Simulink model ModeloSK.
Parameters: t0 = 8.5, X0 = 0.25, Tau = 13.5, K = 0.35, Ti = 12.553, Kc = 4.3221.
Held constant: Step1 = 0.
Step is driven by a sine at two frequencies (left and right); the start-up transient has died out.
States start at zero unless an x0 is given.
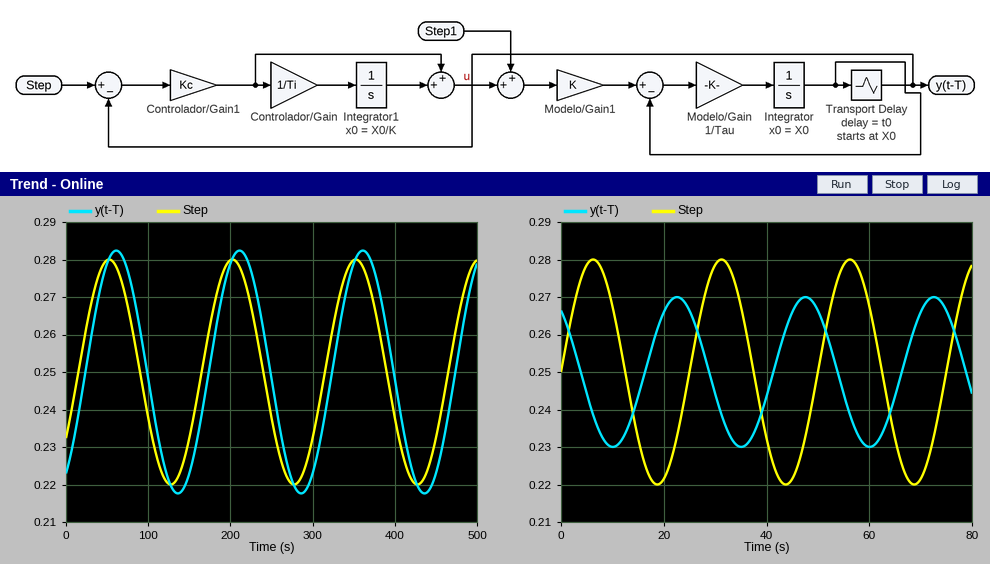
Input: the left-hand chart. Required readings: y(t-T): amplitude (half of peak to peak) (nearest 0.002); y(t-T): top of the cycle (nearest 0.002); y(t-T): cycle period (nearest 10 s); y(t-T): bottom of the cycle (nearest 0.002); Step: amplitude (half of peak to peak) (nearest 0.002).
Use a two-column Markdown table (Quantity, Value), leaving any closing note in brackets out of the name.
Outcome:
| Quantity | Value |
|---|---|
| y(t-T): amplitude (half of peak to peak) | 0.032 |
| y(t-T): top of the cycle | 0.282 |
| y(t-T): cycle period | 150 s |
| y(t-T): bottom of the cycle | 0.218 |
| Step: amplitude (half of peak to peak) | 0.030 |
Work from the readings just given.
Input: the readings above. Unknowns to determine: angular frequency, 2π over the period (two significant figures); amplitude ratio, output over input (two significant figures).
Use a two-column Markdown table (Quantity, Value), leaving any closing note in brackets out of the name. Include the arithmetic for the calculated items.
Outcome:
| Quantity | Value |
|---|---|
| angular frequency, 2π over the period | 2π / 150 = 0.042 rad/s |
| amplitude ratio, output over input | 0.032 / 0.03 = 1.1 |
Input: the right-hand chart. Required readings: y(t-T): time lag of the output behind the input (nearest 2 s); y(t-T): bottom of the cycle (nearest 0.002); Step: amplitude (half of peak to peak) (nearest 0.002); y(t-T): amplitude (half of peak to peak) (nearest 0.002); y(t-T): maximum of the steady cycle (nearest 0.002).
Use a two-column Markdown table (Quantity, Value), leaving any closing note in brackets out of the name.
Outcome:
| Quantity | Value |
|---|---|
| y(t-T): time lag of the output behind the input | 16 s |
| y(t-T): bottom of the cycle | 0.230 |
| Step: amplitude (half of peak to peak) | 0.030 |
| y(t-T): amplitude (half of peak to peak) | 0.020 |
| y(t-T): maximum of the steady cycle | 0.270 |
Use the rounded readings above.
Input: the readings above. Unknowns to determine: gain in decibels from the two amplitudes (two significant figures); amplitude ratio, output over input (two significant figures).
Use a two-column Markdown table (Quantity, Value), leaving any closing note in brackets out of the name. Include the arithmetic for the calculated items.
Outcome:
| Quantity | Value |
|---|---|
| gain in decibels from the two amplitudes | 20 log10(0.02 / 0.03) = -3.5 dB |
| amplitude ratio, output over input | 0.02 / 0.03 = 0.67 |
